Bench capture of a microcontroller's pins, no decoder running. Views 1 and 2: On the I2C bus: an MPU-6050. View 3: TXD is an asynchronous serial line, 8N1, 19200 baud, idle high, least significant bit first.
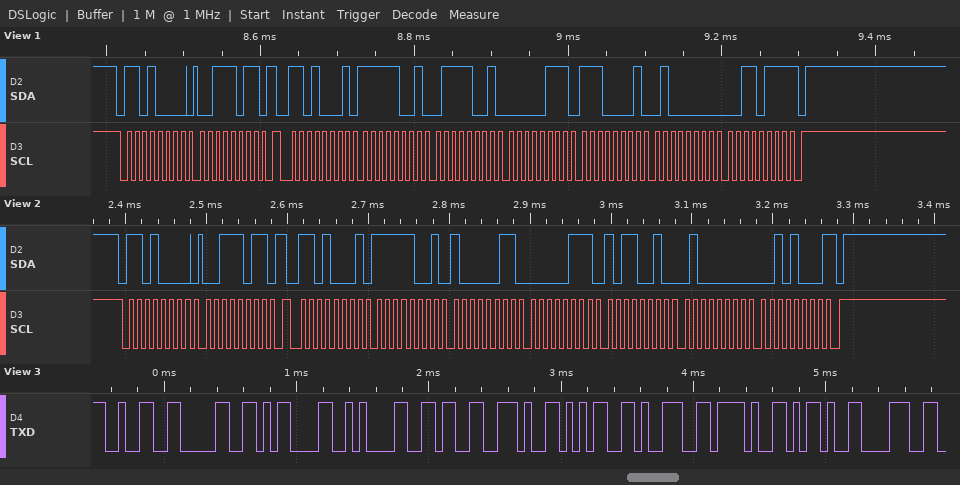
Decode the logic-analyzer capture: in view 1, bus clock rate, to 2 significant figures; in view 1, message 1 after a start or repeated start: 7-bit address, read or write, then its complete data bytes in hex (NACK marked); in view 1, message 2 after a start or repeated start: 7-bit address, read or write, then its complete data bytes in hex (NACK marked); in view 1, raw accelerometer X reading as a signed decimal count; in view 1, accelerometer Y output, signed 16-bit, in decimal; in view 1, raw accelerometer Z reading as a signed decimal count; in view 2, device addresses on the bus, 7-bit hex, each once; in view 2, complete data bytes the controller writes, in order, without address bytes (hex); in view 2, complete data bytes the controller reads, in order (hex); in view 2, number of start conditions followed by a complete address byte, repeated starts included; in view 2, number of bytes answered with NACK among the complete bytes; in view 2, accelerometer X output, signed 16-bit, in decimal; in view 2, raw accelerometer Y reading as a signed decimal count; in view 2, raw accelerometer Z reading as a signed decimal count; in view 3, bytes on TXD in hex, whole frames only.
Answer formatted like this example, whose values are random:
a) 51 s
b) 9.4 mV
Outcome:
a) 100 kHz
b) 0x68 write: 3B
c) 0x68 read: F9 79 07 E1 40 37 NACK
d) -1671
e) 2017
f) 16439
g) 0x68
h) 3B
i) F9 83 07 B2 40 28
j) 2
k) 1
l) -1661
m) 1970
n) 16424
o) 32 30 0D 0A 36 2E 35 39 2F 2D 38
